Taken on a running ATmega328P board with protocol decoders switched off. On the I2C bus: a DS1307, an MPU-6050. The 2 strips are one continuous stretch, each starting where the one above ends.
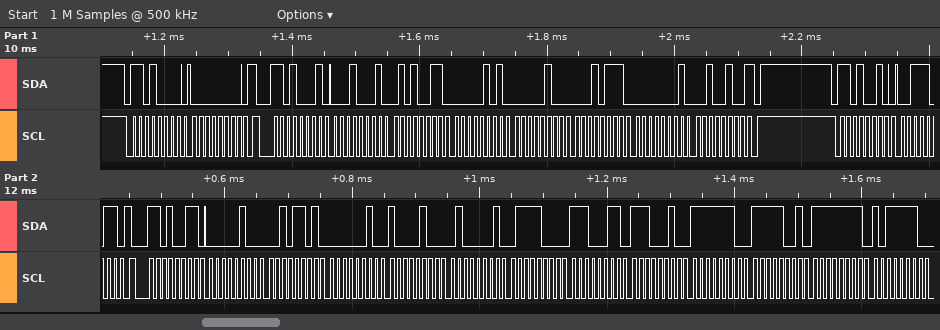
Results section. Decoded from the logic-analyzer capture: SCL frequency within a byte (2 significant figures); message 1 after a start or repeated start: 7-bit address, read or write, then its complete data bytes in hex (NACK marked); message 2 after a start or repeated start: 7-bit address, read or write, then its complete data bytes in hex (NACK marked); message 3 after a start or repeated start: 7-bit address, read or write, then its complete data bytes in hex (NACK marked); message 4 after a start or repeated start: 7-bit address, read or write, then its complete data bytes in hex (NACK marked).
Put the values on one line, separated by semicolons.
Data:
100 kHz; 0x68 write: 00; 0x68 read: 11 53 05 04 17 01 24 NACK; 0x69 write: 3B; 0x69 read: 04 2D 02 84 41 78 E3 E2 FE F9 FF BE
